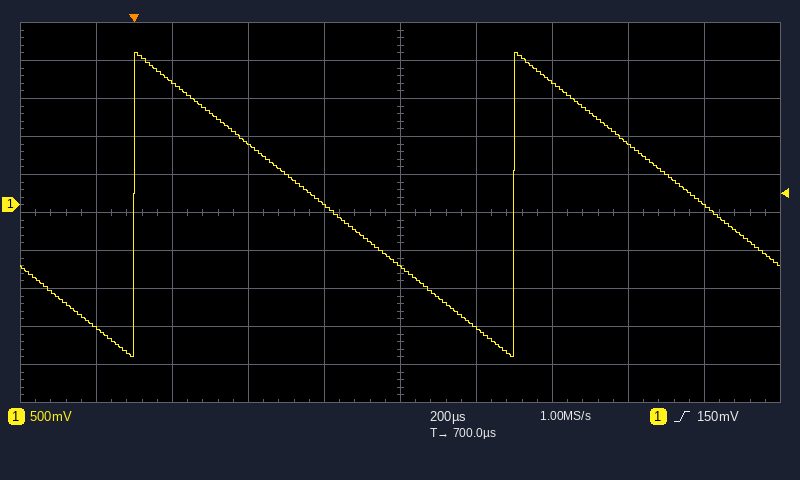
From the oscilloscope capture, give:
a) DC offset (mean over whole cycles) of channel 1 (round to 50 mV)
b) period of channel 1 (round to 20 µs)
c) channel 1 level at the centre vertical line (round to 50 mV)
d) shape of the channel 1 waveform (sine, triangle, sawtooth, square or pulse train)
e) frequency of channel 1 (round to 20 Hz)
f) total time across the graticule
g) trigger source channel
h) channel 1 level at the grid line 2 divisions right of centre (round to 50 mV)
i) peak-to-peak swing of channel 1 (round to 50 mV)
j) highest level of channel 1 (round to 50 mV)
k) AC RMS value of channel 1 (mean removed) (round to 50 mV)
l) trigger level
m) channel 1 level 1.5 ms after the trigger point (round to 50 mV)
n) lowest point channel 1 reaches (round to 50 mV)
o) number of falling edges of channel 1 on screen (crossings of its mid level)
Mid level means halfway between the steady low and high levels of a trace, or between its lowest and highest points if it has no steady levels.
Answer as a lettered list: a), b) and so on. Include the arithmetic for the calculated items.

a) (2.00 V + (-2.00 V)) / 2 ≈ 0 mV
b) 1.00 ms
c) -800 mV
d) sawtooth
e) 1 / 1.00 ms ≈ 1.00 kHz
f) 2 ms
g) channel 1
h) 1.60 V
i) 2.00 V − (-2.00 V) = 4.00 V
j) 2.00 V
k) 4.00 V / (2√3) ≈ 1.15 V
l) 150 mV
m) 0 mV
n) -2.00 V
o) 2
